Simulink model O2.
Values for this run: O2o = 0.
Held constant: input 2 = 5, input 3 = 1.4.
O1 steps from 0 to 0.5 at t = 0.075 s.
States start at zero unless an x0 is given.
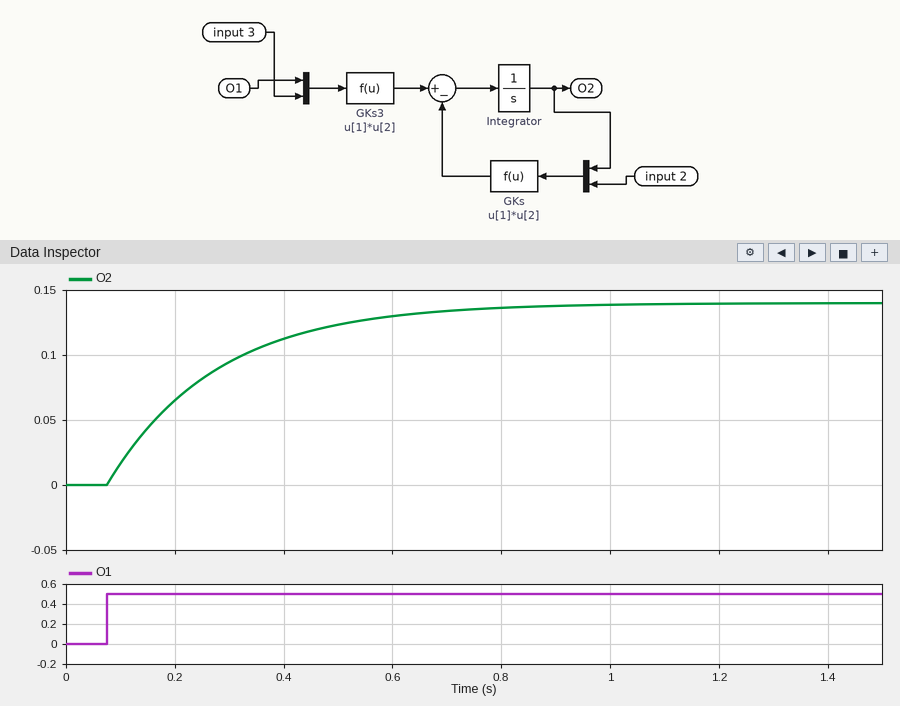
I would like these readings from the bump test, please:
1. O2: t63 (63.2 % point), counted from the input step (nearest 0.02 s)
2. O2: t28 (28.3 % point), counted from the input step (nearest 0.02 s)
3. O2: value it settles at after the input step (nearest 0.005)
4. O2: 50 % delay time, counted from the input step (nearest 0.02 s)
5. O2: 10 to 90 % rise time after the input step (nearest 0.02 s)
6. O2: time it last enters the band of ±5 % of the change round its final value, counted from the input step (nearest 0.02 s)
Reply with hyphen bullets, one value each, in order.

- 0.20 s
- 0.06 s
- 0.140
- 0.14 s
- 0.44 s
- 0.60 s
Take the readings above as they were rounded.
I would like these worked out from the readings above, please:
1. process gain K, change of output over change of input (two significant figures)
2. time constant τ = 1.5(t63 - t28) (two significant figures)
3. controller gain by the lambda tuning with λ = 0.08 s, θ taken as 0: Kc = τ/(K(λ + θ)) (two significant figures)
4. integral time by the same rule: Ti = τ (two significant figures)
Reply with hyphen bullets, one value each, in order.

- 0.28
- 0.21 s
- 9.4
- 0.21 s
